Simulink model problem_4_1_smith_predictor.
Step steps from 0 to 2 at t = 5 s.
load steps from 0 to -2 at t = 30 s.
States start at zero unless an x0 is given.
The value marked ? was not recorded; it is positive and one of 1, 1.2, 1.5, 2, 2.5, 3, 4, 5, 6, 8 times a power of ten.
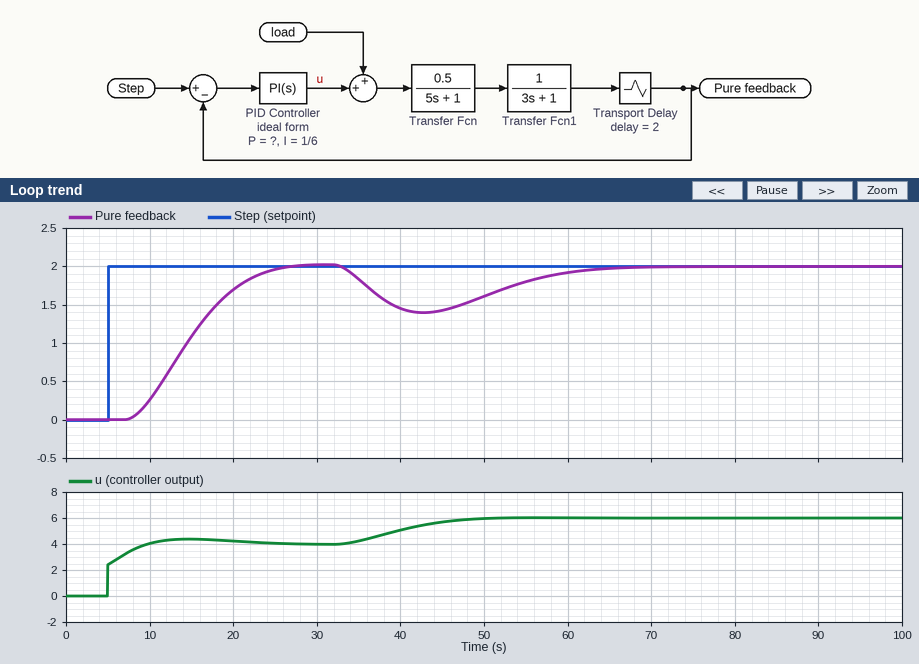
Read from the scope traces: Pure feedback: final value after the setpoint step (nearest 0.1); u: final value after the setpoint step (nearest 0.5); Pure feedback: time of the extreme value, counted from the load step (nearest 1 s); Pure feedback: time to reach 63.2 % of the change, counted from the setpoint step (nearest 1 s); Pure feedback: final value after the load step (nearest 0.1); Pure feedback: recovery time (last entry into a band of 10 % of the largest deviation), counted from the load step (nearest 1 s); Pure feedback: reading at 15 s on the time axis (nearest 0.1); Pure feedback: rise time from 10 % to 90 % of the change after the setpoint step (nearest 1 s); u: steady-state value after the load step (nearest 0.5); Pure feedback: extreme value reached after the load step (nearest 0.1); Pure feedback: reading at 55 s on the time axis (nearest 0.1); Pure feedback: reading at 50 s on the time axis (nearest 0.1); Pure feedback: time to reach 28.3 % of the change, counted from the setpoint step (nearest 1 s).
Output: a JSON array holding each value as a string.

["2.0", "4.0", "13 s", "11 s", "2.0", "31 s", "1.1", "12 s", "6.0", "1.4", "1.8", "1.6", "7 s"]
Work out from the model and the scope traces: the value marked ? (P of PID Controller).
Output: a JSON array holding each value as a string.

["1.2"]
